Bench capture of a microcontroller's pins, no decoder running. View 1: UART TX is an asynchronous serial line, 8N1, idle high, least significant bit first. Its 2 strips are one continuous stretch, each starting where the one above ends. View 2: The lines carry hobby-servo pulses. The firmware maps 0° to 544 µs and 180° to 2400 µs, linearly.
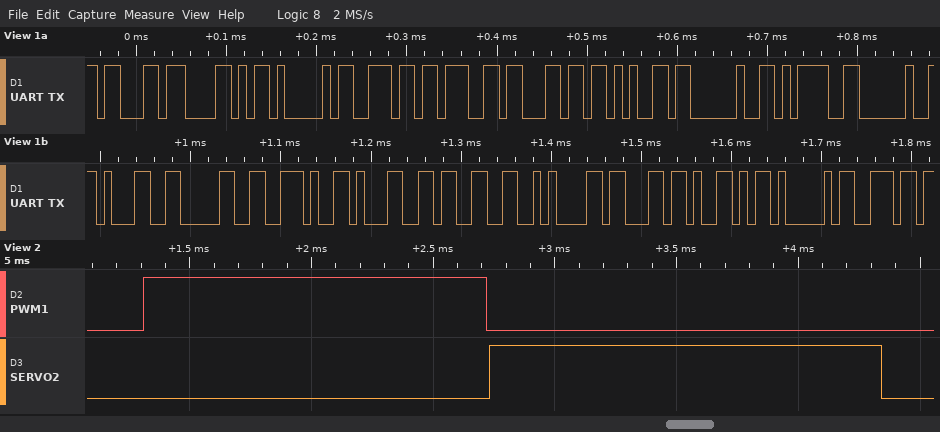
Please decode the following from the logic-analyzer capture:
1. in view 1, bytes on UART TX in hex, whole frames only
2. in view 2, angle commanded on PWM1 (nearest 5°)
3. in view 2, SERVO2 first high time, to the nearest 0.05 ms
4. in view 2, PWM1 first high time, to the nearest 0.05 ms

63 58 41 6E 67 6C 65 20 3D 20 31 30 2E 31 33 0A 63 59 41 6E
85°
1.60 ms
1.40 ms
